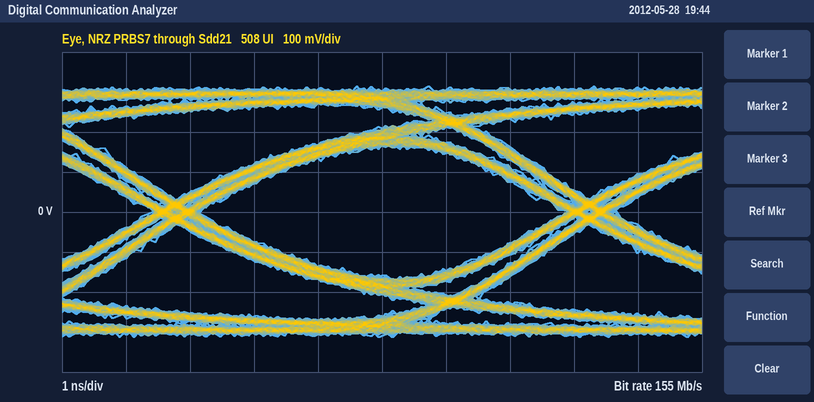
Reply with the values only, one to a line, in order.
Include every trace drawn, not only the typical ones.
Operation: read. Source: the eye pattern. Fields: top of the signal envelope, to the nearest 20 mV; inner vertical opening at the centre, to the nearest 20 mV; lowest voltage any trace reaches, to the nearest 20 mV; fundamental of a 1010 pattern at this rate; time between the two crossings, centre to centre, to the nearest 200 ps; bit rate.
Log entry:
320 mV
320 mV
-320 mV
77.5 MHz
6.4 ns
155 Mb/s
